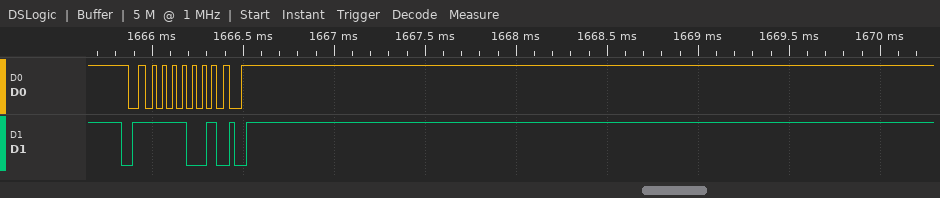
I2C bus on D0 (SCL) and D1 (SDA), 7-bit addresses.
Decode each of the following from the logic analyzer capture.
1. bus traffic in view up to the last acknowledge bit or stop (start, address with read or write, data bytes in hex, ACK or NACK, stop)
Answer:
start, address 7C read ACK, stop
